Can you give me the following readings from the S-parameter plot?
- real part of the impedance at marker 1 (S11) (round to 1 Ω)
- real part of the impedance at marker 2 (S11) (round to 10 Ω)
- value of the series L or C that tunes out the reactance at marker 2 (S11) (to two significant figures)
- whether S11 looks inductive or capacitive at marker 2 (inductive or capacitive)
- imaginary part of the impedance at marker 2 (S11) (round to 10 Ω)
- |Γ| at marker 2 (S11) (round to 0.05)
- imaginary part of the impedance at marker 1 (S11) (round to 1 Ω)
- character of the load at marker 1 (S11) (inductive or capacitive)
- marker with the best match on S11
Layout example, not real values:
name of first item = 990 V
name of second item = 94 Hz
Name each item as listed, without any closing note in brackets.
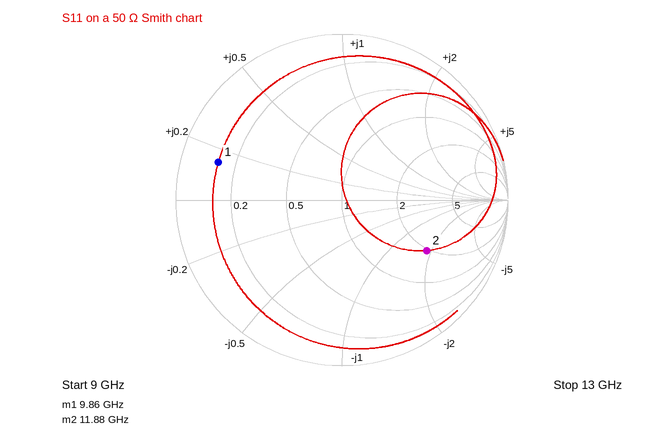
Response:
real part of the impedance at marker 1 (S11) = 6 Ω
real part of the impedance at marker 2 (S11) = 100 Ω
value of the series L or C that tunes out the reactance at marker 2 (S11) = 1.2 nH
whether S11 looks inductive or capacitive at marker 2 = capacitive
imaginary part of the impedance at marker 2 (S11) = -90 Ω
|Γ| at marker 2 (S11) = 0.60
imaginary part of the impedance at marker 1 (S11) = +7 Ω
character of the load at marker 1 (S11) = inductive
marker with the best match on S11 = marker 2
